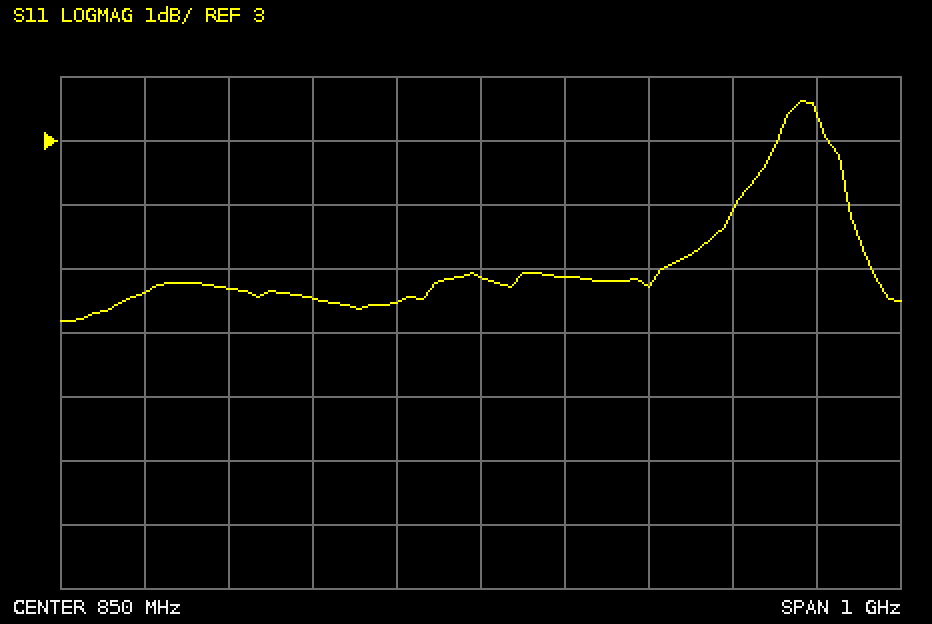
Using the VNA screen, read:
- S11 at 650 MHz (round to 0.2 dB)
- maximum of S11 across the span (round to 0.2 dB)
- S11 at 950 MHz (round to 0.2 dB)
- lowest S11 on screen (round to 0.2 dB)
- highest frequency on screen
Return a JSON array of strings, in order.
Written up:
["0.6 dB", "3.6 dB", "0.8 dB", "0.2 dB", "1.35 GHz"]
